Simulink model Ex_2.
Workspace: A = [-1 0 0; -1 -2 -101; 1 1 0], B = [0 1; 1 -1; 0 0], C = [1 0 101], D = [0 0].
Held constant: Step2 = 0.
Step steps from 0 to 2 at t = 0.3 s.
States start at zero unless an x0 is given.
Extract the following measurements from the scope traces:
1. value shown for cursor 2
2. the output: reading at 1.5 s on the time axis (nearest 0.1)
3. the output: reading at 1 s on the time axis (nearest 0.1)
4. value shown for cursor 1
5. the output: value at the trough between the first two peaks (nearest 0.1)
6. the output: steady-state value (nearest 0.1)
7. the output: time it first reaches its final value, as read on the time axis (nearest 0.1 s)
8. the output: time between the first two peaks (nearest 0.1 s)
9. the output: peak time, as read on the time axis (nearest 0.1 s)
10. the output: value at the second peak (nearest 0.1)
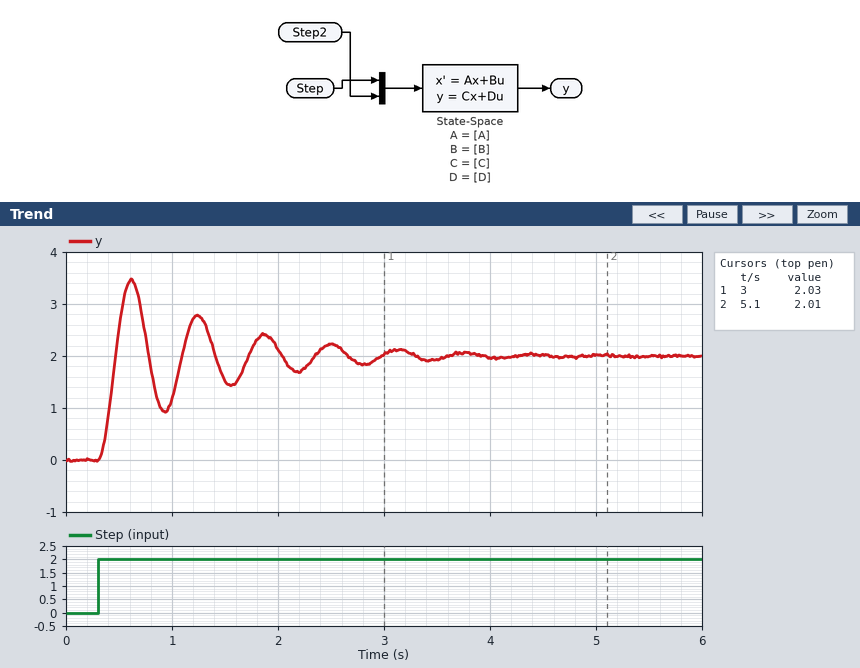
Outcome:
2.01
1.5
1.2
2.03
0.9
2.0
0.5 s
0.6 s
0.6 s
2.8
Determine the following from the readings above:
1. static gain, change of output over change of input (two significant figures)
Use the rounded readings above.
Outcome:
1.0
